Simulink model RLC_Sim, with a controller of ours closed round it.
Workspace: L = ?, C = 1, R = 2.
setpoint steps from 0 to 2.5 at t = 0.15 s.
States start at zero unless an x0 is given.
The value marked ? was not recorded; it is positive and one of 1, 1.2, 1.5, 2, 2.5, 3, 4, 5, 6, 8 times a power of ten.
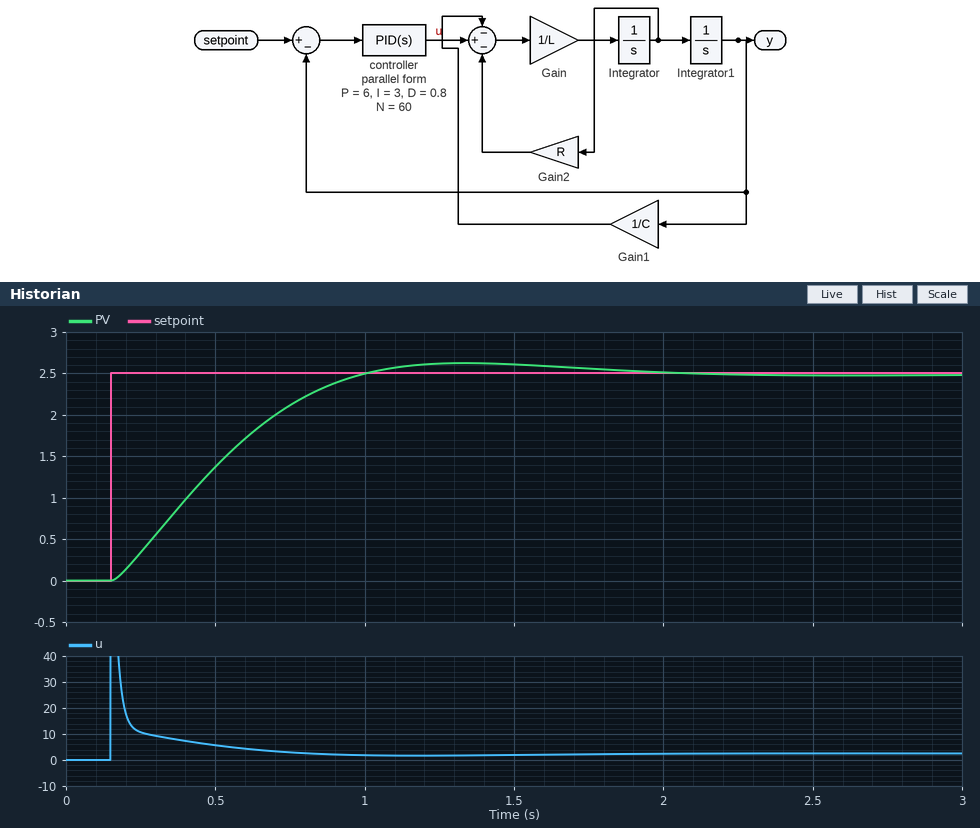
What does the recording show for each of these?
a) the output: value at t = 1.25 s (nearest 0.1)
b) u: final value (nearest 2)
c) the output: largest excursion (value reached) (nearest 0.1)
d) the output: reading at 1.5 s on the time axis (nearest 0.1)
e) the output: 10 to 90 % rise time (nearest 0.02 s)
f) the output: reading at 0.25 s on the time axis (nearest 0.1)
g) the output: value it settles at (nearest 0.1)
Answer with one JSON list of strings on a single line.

["2.6", "2", "2.6", "2.6", "0.58 s", "0.3", "2.5"]
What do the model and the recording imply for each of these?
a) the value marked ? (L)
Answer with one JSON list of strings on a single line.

["0.6"]
